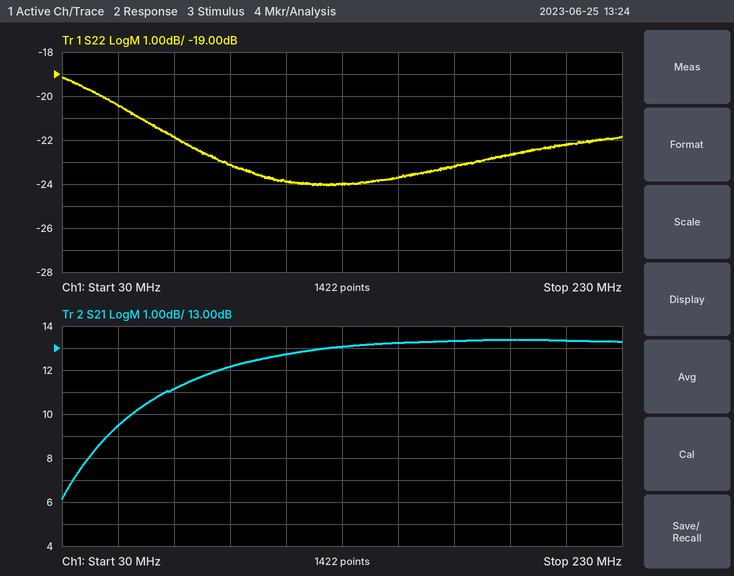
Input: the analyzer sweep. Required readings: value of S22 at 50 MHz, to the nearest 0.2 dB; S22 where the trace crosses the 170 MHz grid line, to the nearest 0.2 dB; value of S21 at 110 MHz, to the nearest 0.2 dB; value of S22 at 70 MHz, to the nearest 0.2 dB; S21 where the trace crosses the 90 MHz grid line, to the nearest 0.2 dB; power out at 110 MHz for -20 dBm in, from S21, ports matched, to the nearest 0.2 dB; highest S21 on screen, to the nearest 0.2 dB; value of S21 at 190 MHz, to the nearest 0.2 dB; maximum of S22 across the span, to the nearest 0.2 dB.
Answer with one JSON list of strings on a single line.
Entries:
["-20.4 dB", "-23.2 dB", "12.8 dB", "-21.8 dB", "12.2 dB", "-7.2 dBm", "13.4 dB", "13.4 dB", "-19.2 dB"]
